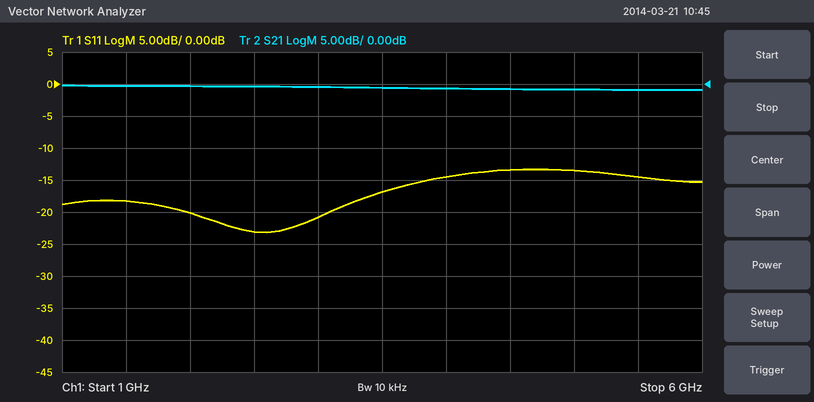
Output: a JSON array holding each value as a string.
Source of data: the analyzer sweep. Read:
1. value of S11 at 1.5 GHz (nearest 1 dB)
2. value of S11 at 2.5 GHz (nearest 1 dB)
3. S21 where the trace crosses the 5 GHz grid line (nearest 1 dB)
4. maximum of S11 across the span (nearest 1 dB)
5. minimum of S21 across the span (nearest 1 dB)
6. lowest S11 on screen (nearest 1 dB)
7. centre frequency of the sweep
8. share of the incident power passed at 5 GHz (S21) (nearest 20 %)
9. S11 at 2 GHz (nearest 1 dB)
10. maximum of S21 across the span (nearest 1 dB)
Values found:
["-18 dB", "-23 dB", "-1 dB", "-13 dB", "-1 dB", "-23 dB", "3.5 GHz", "80 %", "-20 dB", "0 dB"]
